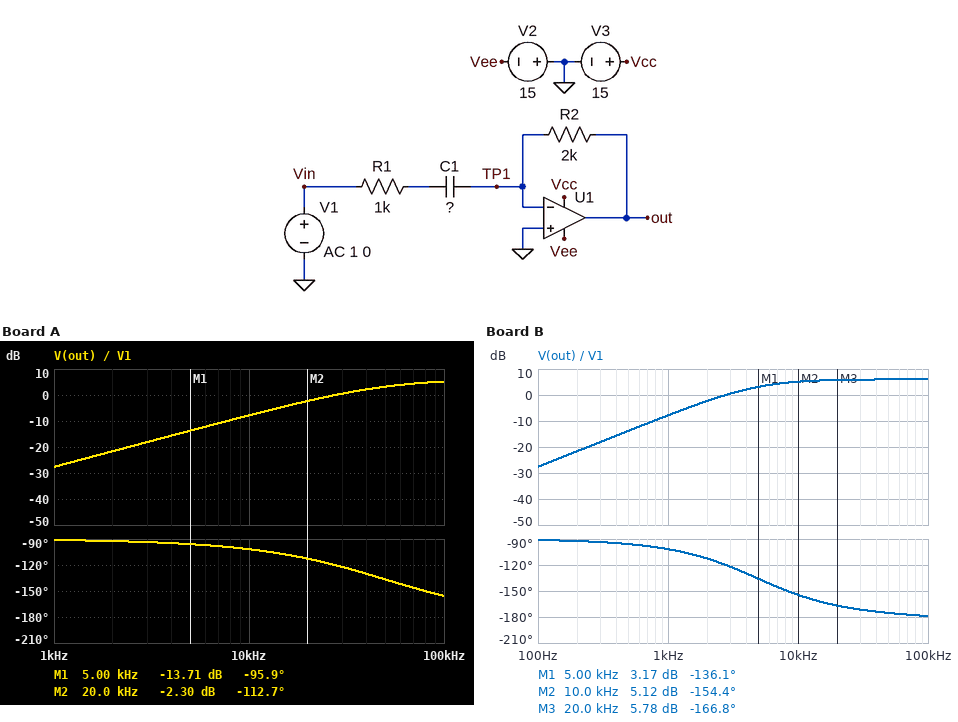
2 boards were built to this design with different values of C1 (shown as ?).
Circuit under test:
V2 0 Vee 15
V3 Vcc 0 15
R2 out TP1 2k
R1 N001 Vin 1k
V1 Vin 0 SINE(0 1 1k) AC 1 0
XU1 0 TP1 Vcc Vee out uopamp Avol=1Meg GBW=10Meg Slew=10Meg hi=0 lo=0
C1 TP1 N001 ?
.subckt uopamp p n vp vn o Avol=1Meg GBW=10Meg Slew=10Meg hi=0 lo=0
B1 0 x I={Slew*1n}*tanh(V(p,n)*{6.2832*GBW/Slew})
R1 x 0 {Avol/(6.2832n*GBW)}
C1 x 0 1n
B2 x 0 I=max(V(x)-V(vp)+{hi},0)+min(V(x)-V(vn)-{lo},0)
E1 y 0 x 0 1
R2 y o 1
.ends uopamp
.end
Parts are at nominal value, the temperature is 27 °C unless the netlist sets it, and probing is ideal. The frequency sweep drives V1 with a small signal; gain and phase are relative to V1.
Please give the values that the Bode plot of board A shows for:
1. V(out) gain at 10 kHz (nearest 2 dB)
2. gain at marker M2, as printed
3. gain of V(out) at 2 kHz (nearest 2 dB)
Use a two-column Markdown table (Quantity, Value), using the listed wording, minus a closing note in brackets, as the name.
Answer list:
| Quantity | Value |
|---|---|
| V(out) gain at 10 kHz | -8 dB |
| gain at marker M2, as printed | -2.30 dB |
| gain of V(out) at 2 kHz | -22 dB |
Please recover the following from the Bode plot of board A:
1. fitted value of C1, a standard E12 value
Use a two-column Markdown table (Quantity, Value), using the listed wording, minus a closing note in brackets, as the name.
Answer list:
| Quantity | Value |
|---|---|
| fitted value of C1, a standard E12 value | 3.3 nF |
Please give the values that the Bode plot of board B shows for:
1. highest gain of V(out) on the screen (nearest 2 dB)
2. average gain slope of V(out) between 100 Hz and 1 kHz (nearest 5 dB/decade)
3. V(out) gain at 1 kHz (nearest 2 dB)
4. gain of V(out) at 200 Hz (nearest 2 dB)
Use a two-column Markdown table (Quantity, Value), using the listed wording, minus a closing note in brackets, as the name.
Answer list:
| Quantity | Value |
|---|---|
| highest gain of V(out) on the screen | 6 dB |
| average gain slope of V(out) between 100 Hz and 1 kHz | 20 dB/decade |
| V(out) gain at 1 kHz | -8 dB |
| gain of V(out) at 200 Hz | -22 dB |
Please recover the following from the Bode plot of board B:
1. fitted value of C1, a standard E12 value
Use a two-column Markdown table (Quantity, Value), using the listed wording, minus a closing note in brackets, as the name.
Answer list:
| Quantity | Value |
|---|---|
| fitted value of C1, a standard E12 value | 33 nF |
